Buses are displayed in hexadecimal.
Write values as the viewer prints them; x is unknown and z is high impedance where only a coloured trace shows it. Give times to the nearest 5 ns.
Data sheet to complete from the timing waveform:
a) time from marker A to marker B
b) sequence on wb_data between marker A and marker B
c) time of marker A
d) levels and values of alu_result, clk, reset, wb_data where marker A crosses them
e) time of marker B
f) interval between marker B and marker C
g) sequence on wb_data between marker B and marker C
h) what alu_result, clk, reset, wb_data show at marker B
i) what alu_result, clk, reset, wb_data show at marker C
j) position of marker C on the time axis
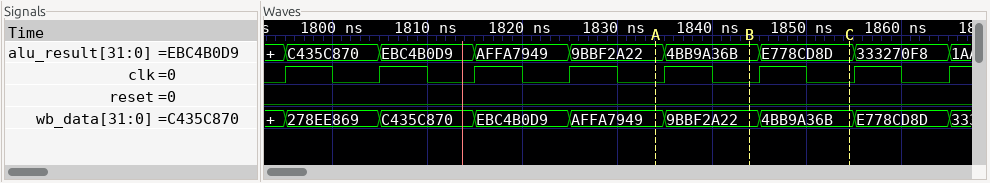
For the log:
10 ns
AFFA7949, 9BBF2A22
1835 ns
alu_result=9BBF2A22, clk=0, reset=0, wb_data=AFFA7949
1845 ns
10 ns
9BBF2A22, 4BB9A36B
alu_result=4BB9A36B, clk=0, reset=0, wb_data=9BBF2A22
alu_result=E778CD8D, clk=0, reset=0, wb_data=4BB9A36B
1855 ns
